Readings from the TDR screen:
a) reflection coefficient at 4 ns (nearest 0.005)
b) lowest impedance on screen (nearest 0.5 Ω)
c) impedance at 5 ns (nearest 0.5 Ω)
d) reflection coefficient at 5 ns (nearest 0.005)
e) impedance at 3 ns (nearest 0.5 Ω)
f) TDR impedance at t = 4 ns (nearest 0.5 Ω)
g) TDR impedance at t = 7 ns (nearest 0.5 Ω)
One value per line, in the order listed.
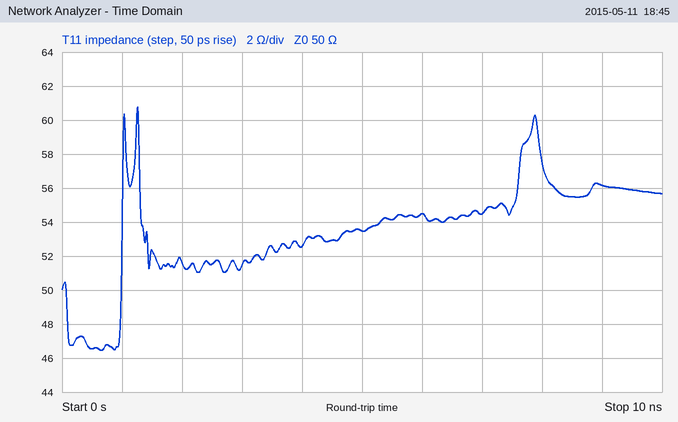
+0.025
46.5 Ω
53.5 Ω
+0.035
51.5 Ω
52.5 Ω
54.5 Ω
